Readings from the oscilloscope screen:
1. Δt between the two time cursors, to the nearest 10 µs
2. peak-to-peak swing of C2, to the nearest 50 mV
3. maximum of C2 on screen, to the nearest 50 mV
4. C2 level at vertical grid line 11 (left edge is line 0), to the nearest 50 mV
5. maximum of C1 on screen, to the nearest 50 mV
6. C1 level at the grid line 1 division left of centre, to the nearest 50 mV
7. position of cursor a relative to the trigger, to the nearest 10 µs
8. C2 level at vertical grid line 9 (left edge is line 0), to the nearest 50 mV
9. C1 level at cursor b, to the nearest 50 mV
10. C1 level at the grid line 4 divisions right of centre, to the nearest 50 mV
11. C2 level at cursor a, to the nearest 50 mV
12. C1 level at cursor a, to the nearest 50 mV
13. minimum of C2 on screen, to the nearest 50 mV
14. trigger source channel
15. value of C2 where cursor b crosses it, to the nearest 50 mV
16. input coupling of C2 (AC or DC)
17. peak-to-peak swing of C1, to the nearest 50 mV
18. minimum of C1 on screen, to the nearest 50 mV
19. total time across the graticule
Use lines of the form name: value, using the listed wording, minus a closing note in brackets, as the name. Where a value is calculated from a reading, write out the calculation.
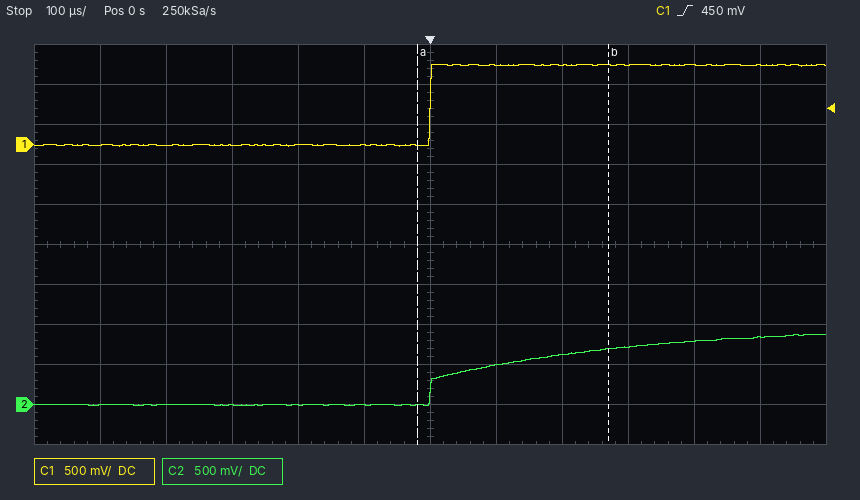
Δt between the two time cursors, to the nearest 10 µs: 290 µs
peak-to-peak swing of C2, to the nearest 50 mV: 900 mV − (0 mV) = 900 mV
maximum of C2 on screen, to the nearest 50 mV: 900 mV
C2 level at vertical grid line 11 (left edge is line 0), to the nearest 50 mV: 850 mV
maximum of C1 on screen, to the nearest 50 mV: 1.00 V
C1 level at the grid line 1 division left of centre, to the nearest 50 mV: 0 mV
position of cursor a relative to the trigger, to the nearest 10 µs: -20 µs
C2 level at vertical grid line 9 (left edge is line 0), to the nearest 50 mV: 700 mV
C1 level at cursor b, to the nearest 50 mV: 1.00 V
C1 level at the grid line 4 divisions right of centre, to the nearest 50 mV: 1.00 V
C2 level at cursor a, to the nearest 50 mV: 0 mV
C1 level at cursor a, to the nearest 50 mV: 0 mV
minimum of C2 on screen, to the nearest 50 mV: 0 mV
trigger source channel: C1
value of C2 where cursor b crosses it, to the nearest 50 mV: 700 mV
input coupling of C2: DC
peak-to-peak swing of C1, to the nearest 50 mV: 1.00 V − (0 mV) = 1.00 V
minimum of C1 on screen, to the nearest 50 mV: 0 mV
total time across the graticule: 1.2 ms
